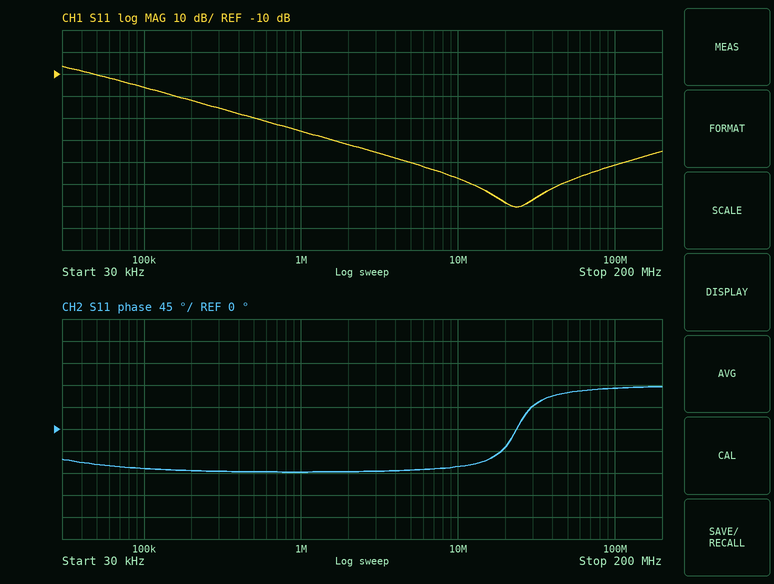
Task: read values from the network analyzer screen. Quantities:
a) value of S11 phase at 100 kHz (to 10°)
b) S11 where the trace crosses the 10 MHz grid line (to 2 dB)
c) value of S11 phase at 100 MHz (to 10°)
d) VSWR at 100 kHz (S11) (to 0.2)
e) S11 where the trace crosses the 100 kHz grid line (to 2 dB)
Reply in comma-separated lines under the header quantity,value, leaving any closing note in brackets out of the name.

quantity,value
value of S11 phase at 100 kHz,-80°
S11 where the trace crosses the 10 MHz grid line,-58 dB
value of S11 phase at 100 MHz,80°
VSWR at 100 kHz (S11),1.4
S11 where the trace crosses the 100 kHz grid line,-16 dB
